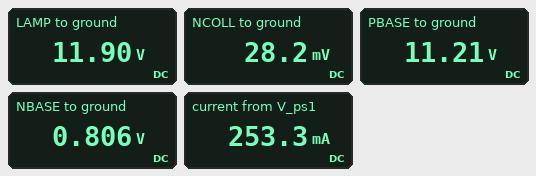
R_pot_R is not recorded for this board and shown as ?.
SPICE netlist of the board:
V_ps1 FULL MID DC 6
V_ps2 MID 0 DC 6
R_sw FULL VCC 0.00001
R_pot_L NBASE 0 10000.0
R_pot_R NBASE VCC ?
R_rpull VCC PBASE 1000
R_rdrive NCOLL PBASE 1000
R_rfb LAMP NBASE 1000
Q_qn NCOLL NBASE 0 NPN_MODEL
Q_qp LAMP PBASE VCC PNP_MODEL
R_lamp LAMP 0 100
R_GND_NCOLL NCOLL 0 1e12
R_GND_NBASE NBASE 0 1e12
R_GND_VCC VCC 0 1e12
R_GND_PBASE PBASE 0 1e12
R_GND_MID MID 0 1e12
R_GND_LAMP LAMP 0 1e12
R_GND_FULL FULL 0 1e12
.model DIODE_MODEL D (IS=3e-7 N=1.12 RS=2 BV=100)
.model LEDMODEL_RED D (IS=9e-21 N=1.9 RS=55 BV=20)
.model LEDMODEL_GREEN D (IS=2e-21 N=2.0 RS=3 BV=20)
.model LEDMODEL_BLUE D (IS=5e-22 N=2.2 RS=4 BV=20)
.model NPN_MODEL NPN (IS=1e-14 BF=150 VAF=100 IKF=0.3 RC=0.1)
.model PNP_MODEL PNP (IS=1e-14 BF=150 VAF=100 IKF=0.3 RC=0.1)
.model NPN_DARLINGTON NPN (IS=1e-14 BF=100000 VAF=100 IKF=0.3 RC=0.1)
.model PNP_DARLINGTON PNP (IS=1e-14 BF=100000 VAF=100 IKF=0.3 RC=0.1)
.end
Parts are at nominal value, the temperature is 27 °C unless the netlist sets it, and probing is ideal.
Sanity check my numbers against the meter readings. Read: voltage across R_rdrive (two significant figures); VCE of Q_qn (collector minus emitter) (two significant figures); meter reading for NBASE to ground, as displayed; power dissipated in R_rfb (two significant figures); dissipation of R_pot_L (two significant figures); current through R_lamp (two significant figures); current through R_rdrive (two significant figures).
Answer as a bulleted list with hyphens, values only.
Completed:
- 11 V
- 28 mV
- 0.806 V
- 120 mW
- 65 µW
- 120 mA
- 11 mA
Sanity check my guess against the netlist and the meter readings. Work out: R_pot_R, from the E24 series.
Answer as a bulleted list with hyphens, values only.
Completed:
- 100 Ω
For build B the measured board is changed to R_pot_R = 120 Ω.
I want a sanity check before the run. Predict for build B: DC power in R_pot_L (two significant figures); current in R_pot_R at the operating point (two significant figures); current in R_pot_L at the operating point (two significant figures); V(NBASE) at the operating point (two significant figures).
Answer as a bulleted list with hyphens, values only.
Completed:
- 64 µW
- 93 mA
- 80 µA
- 800 mV
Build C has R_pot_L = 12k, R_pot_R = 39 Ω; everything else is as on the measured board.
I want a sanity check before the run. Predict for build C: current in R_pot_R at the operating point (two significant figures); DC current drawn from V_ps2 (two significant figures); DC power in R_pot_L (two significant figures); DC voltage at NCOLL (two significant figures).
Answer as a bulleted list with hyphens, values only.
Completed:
- 290 mA
- 430 mA
- 58 µW
- 34 mV
